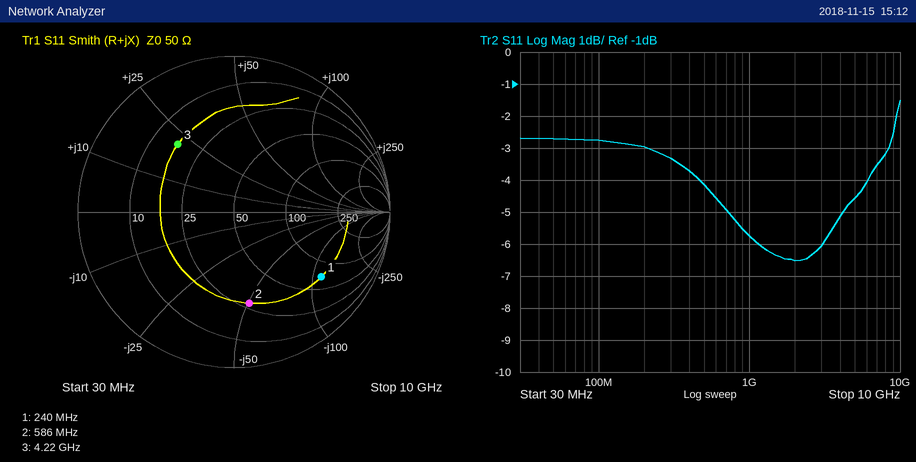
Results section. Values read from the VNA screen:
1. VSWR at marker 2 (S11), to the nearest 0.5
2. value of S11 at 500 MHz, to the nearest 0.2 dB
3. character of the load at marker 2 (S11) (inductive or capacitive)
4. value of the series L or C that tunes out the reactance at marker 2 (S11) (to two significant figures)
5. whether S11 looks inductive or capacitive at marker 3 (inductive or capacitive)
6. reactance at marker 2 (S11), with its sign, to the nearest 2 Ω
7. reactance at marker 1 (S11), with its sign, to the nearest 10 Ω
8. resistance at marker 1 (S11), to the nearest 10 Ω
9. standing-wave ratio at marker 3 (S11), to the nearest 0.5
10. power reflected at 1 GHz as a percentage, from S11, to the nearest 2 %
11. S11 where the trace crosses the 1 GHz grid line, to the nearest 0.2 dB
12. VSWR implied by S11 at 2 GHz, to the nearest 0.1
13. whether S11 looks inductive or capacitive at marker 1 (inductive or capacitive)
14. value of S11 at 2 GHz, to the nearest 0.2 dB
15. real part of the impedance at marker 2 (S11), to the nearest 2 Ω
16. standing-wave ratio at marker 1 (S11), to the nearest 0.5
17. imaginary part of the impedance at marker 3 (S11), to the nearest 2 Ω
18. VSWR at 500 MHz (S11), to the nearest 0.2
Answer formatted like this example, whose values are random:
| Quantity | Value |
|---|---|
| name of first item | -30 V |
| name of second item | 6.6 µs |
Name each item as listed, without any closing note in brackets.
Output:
| Quantity | Value |
|---|---|
| VSWR at marker 2 (S11), to the nearest 0.5 | 4.0 |
| value of S11 at 500 MHz, to the nearest 0.2 dB | -4.2 dB |
| character of the load at marker 2 (S11) | capacitive |
| value of the series L or C that tunes out the reactance at marker 2 (S11) | 14 nH |
| whether S11 looks inductive or capacitive at marker 3 | inductive |
| reactance at marker 2 (S11), with its sign, to the nearest 2 Ω | -50 Ω |
| reactance at marker 1 (S11), with its sign, to the nearest 10 Ω | -110 Ω |
| resistance at marker 1 (S11), to the nearest 10 Ω | 70 Ω |
| standing-wave ratio at marker 3 (S11), to the nearest 0.5 | 3.5 |
| power reflected at 1 GHz as a percentage, from S11, to the nearest 2 % | 26 % |
| S11 where the trace crosses the 1 GHz grid line, to the nearest 0.2 dB | -5.8 dB |
| VSWR implied by S11 at 2 GHz, to the nearest 0.1 | 2.8 |
| whether S11 looks inductive or capacitive at marker 1 | capacitive |
| value of S11 at 2 GHz, to the nearest 0.2 dB | -6.6 dB |
| real part of the impedance at marker 2 (S11), to the nearest 2 Ω | 28 Ω |
| standing-wave ratio at marker 1 (S11), to the nearest 0.5 | 5.5 |
| imaginary part of the impedance at marker 3 (S11), to the nearest 2 Ω | +22 Ω |
| VSWR at 500 MHz (S11), to the nearest 0.2 | 4.2 |
